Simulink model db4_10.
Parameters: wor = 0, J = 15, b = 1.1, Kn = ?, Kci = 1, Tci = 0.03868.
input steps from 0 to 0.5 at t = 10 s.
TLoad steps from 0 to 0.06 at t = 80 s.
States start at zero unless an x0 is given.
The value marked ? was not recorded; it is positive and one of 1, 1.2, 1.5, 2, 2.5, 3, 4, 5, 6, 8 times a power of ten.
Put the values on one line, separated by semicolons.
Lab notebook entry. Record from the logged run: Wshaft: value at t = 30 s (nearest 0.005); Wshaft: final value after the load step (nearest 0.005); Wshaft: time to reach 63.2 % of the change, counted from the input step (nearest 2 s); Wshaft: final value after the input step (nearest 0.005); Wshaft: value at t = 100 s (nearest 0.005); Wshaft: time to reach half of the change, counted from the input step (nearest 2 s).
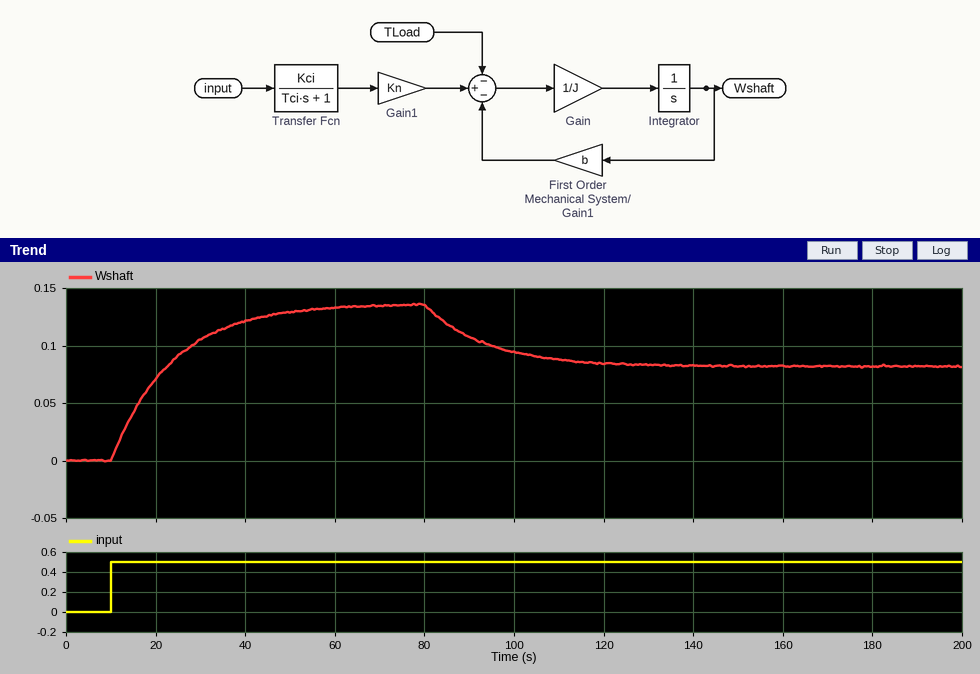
0.105; 0.080; 14 s; 0.135; 0.095; 10 s
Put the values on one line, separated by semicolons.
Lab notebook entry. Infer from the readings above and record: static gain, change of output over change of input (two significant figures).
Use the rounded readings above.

0.27
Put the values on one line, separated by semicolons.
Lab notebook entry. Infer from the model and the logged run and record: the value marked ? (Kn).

0.3
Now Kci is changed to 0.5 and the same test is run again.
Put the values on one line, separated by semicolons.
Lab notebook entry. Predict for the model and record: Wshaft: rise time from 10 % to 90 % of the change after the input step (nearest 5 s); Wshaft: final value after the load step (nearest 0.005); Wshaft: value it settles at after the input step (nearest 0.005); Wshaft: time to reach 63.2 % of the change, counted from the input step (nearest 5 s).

30 s; 0.015; 0.070; 15 s
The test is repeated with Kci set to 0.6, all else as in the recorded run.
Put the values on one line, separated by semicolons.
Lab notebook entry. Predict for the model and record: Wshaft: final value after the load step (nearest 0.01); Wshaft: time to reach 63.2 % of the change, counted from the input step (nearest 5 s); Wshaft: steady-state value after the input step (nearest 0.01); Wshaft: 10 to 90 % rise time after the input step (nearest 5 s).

0.03; 15 s; 0.08; 30 s
